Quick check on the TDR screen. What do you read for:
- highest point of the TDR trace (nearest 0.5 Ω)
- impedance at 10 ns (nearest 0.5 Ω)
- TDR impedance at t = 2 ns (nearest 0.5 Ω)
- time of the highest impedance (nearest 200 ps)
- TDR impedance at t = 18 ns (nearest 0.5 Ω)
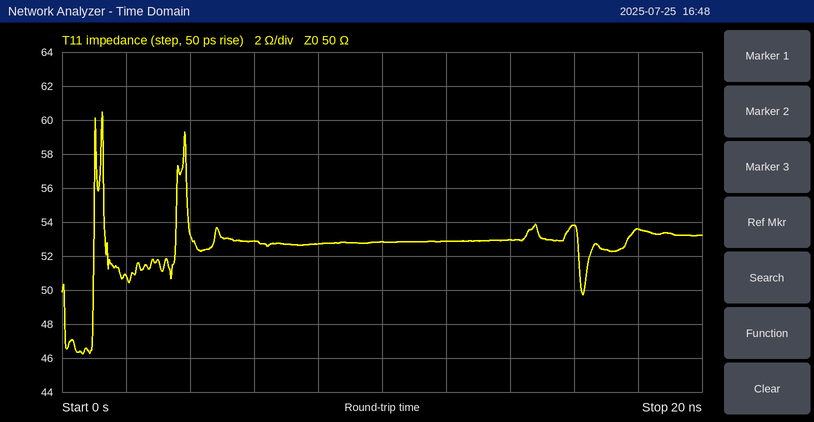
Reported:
60.5 Ω
53.0 Ω
51.0 Ω
1.2 ns
53.5 Ω
